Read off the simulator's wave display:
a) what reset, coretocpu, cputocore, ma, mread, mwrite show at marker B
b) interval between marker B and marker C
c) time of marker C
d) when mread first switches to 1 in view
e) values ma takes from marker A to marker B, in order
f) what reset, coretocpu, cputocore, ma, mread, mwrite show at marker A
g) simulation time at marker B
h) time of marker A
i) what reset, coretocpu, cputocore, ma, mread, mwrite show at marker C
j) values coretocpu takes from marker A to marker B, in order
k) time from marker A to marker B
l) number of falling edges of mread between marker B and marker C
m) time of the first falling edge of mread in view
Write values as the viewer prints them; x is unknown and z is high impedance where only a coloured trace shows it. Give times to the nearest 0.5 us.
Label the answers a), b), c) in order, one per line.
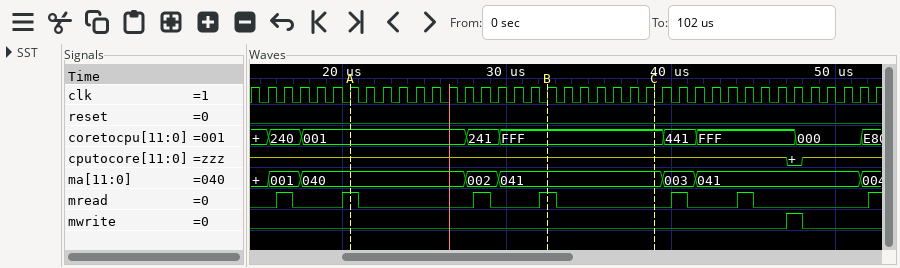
a) reset=0, coretocpu=FFF, cputocore=z, ma=041, mread=1, mwrite=0
b) 6.5 us
c) 39 us
d) 16 us
e) 040, 002, 041
f) reset=0, coretocpu=001, cputocore=z, ma=040, mread=1, mwrite=0
g) 32.5 us
h) 20.5 us
i) reset=0, coretocpu=FFF, cputocore=z, ma=041, mread=0, mwrite=0
j) 001, 241, FFF
k) 12 us
l) 1
m) 17 us
